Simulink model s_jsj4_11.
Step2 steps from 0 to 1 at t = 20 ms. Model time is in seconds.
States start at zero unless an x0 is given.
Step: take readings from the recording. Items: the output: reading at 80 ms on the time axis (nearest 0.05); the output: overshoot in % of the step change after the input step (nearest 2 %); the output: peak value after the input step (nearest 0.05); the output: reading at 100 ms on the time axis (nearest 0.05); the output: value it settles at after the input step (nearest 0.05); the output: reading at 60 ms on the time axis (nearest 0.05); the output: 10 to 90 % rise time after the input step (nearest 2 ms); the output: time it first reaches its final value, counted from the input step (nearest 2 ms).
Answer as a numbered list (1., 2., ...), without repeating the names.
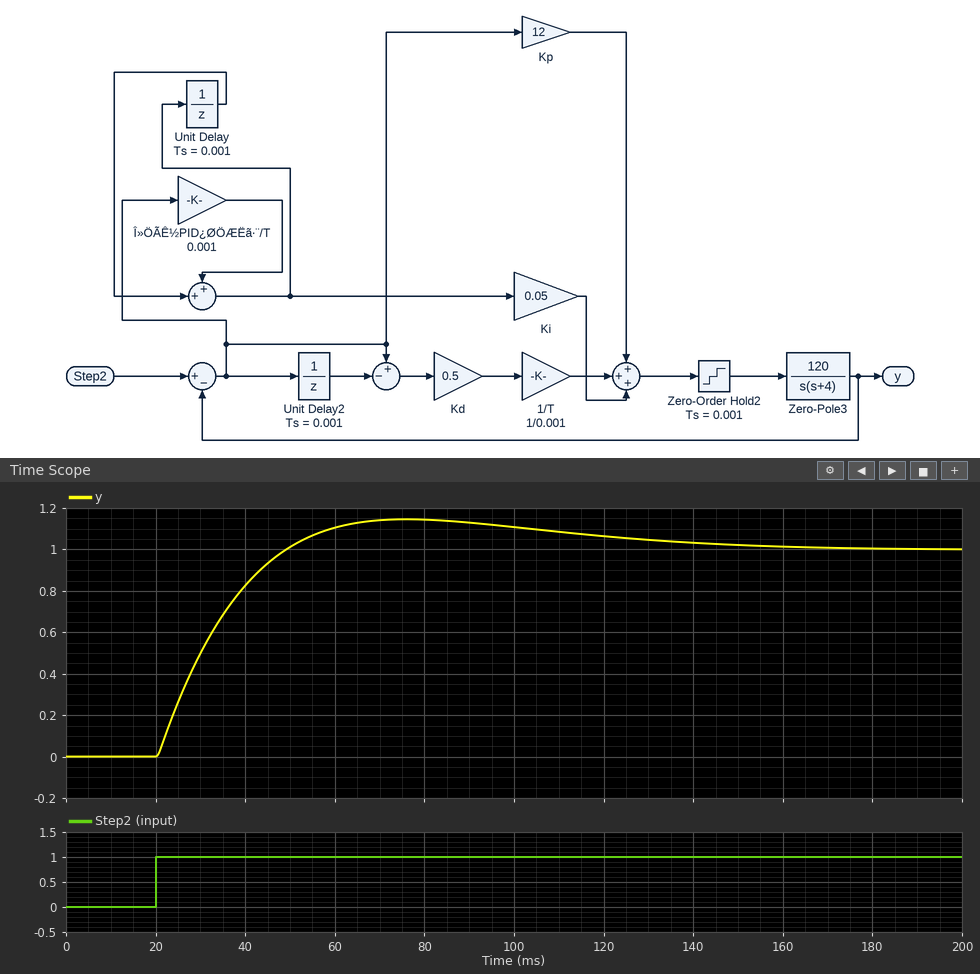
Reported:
1. 1.15
2. 14 %
3. 1.15
4. 1.10
5. 1.00
6. 1.10
7. 22 ms
8. 30 ms
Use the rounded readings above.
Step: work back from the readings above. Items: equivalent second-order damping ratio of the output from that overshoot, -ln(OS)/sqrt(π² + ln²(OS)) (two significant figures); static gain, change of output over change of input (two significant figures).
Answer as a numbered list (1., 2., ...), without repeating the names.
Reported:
1. 0.53
2. 1.0
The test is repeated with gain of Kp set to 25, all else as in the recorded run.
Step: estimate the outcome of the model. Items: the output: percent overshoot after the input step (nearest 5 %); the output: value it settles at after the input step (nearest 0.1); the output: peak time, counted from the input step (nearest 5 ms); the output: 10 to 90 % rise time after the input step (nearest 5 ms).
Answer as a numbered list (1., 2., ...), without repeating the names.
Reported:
1. 25 %
2. 1.0
3. 40 ms
4. 15 ms
